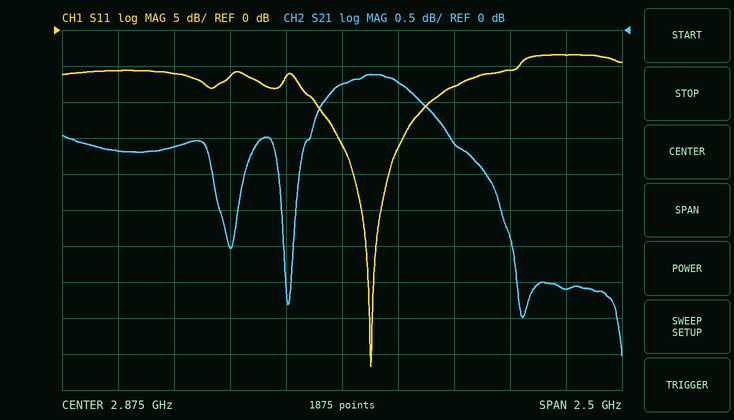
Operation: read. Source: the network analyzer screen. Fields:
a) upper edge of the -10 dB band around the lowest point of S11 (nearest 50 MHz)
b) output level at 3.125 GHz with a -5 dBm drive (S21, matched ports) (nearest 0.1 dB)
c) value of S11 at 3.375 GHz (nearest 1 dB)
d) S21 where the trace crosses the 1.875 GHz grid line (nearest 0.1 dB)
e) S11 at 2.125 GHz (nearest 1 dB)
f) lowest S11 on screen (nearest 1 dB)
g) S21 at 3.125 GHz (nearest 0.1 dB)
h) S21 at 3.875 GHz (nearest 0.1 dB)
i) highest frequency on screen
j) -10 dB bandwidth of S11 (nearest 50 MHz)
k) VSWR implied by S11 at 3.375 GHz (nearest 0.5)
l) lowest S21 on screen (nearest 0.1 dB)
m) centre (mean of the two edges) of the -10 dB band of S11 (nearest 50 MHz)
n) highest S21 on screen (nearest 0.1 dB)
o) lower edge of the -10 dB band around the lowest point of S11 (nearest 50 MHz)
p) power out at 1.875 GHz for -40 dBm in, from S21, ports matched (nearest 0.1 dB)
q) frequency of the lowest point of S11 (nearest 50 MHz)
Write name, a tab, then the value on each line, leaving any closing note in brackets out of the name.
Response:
upper edge of the -10 dB band around the lowest point of S11	3.25 GHz
output level at 3.125 GHz with a -5 dBm drive (S21, matched ports)	-5.7 dBm
value of S11 at 3.375 GHz	-8 dB
S21 where the trace crosses the 1.875 GHz grid line	-1.7 dB
S11 at 2.125 GHz	-6 dB
lowest S11 on screen	-47 dB
S21 at 3.125 GHz	-0.7 dB
S21 at 3.875 GHz	-3.6 dB
highest frequency on screen	4.125 GHz
-10 dB bandwidth of S11	500 MHz
VSWR implied by S11 at 3.375 GHz	2.5
lowest S21 on screen	-4.5 dB
centre (mean of the two edges) of the -10 dB band of S11	3.00 GHz
highest S21 on screen	-0.6 dB
lower edge of the -10 dB band around the lowest point of S11	2.75 GHz
power out at 1.875 GHz for -40 dBm in, from S21, ports matched	-41.7 dBm
frequency of the lowest point of S11	3.00 GHz
